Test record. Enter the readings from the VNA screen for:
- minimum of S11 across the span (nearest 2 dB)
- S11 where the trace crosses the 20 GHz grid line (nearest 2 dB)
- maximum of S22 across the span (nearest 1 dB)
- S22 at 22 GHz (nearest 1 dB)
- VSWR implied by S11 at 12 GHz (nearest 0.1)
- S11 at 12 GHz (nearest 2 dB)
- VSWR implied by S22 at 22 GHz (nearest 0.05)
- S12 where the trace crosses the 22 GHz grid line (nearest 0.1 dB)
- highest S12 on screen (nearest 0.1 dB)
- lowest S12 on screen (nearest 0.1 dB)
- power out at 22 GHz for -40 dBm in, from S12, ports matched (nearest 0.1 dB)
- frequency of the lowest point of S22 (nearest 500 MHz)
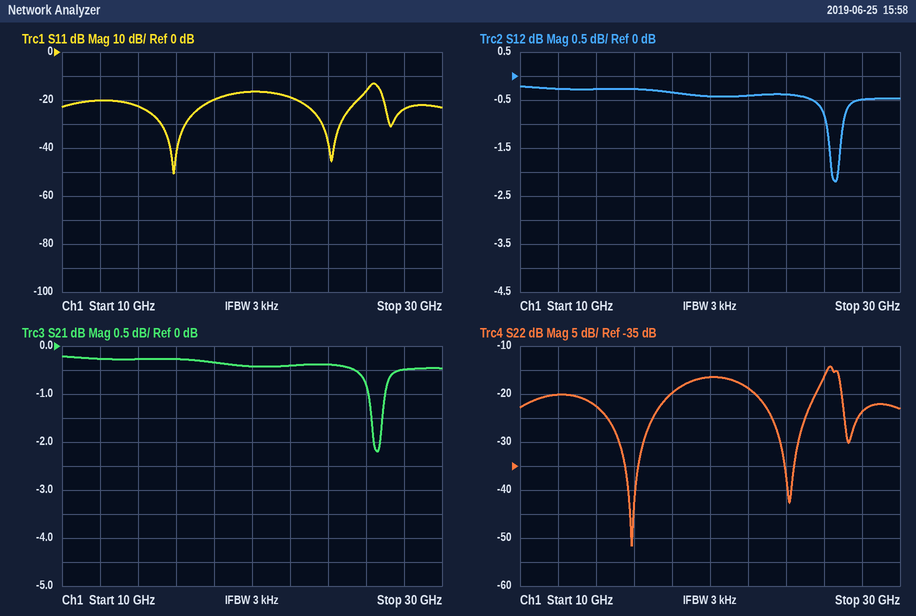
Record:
-50 dB
-16 dB
-14 dB
-19 dB
1.2
-20 dB
1.25
-0.4 dB
-0.2 dB
-2.2 dB
-40.4 dBm
16.0 GHz
